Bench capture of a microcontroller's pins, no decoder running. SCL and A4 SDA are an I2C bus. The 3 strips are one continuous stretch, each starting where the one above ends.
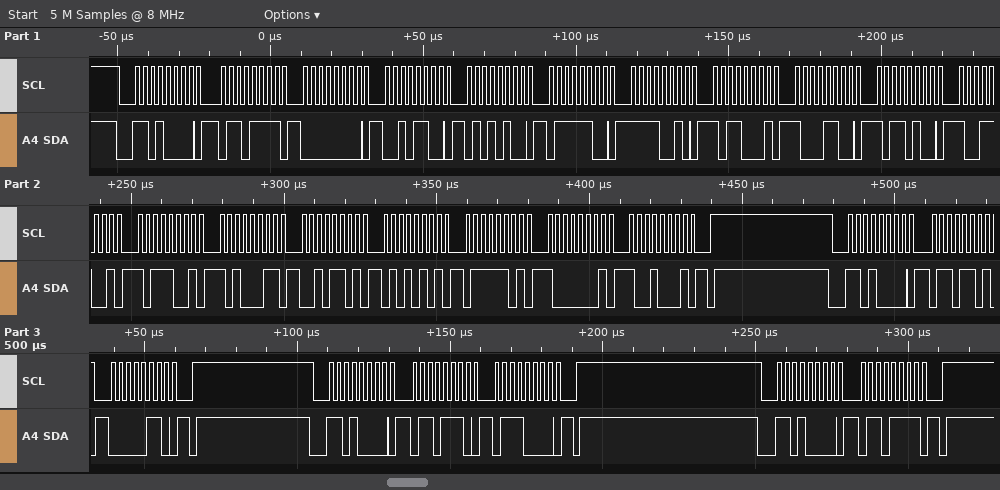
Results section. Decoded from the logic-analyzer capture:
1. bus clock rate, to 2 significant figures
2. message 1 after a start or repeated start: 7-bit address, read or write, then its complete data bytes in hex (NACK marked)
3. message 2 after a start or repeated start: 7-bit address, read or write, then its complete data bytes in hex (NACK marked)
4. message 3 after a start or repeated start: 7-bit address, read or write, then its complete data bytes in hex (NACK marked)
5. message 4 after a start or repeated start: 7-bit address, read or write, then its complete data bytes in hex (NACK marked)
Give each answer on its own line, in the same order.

400 kHz
0x68 write: 6F 00 2C 54 7C F2 B1 8C B4 99 B9 A3 2D 55 7D 81 91
0x68 write: 6D 06
0x68 write: 6E 70
0x68 write: 6F
